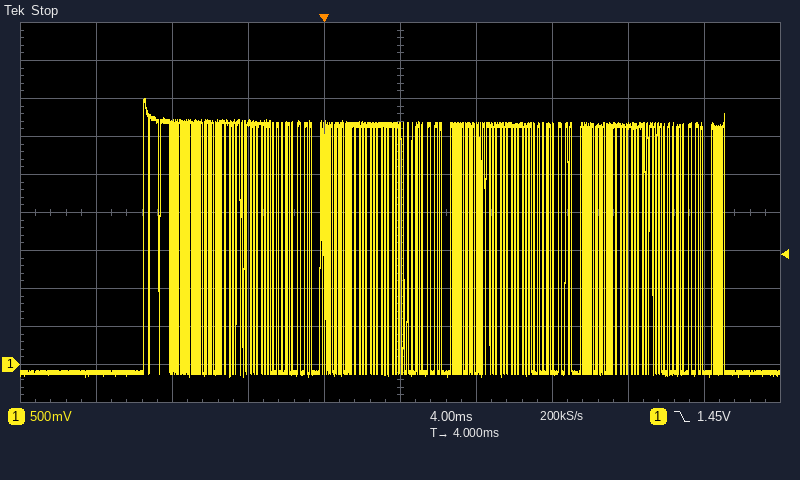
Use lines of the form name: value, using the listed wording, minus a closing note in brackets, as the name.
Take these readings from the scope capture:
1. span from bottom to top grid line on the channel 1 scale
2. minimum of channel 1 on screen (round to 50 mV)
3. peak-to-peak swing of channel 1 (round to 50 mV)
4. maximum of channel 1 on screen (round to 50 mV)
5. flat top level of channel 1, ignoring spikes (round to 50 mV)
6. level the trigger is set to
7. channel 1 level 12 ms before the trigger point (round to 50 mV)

span from bottom to top grid line on the channel 1 scale: 5 V
minimum of channel 1 on screen: -150 mV
peak-to-peak swing of channel 1: 3.65 V
maximum of channel 1 on screen: 3.50 V
flat top level of channel 1, ignoring spikes: 3.15 V
level the trigger is set to: 1.45 V
channel 1 level 12 ms before the trigger point: -100 mV
